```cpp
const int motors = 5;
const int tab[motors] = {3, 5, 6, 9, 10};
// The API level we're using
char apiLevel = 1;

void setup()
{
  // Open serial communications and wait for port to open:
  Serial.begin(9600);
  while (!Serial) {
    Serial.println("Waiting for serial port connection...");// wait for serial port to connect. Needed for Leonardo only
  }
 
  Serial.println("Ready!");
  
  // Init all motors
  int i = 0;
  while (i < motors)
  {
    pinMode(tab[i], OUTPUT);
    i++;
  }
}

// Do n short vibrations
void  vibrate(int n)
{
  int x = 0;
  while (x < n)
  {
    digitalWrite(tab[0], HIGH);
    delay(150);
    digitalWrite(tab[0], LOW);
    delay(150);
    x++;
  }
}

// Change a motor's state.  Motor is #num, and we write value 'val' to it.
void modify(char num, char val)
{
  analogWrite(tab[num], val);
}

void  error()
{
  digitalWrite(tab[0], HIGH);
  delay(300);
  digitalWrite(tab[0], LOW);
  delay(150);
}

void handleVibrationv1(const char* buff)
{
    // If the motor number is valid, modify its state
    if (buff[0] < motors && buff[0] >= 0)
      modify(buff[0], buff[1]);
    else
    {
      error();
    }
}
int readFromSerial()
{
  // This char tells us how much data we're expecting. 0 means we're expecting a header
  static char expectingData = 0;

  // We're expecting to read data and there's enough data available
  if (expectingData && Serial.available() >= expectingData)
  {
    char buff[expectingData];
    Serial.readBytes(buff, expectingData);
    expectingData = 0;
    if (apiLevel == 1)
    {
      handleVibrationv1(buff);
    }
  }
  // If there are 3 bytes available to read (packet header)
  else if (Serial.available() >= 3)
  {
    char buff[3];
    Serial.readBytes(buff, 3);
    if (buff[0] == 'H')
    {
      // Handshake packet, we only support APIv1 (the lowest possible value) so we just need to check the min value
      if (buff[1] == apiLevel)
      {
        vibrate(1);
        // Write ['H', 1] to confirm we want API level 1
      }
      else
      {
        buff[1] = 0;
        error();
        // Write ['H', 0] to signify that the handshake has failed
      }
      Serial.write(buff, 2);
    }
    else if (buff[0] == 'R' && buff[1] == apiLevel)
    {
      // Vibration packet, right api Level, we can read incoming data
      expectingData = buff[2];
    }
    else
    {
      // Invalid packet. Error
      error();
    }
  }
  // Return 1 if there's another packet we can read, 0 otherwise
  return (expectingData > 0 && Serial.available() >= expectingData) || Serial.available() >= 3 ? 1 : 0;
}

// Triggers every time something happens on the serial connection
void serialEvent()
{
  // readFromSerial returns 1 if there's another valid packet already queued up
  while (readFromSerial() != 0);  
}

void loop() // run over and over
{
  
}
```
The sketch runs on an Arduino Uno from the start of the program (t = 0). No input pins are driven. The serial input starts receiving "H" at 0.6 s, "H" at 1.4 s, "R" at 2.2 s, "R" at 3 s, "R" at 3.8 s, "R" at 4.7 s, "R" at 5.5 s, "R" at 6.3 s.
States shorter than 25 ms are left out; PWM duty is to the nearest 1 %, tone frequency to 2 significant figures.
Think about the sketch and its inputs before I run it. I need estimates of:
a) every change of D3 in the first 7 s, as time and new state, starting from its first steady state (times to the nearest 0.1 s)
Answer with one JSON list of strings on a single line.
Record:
["0 s low; 2.2 s high; 2.5 s low; 4.7 s high; 5 s low"]
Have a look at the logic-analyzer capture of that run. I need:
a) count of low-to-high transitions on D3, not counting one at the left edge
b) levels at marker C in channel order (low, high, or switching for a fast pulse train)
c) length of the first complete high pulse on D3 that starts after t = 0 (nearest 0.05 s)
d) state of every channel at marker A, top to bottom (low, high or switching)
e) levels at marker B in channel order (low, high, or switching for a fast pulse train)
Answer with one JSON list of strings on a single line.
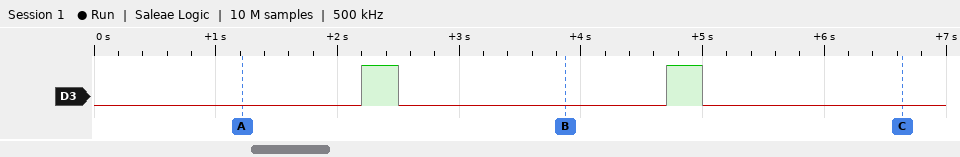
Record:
["2", "D3 low", "0.30 s", "D3 low", "D3 low"]
